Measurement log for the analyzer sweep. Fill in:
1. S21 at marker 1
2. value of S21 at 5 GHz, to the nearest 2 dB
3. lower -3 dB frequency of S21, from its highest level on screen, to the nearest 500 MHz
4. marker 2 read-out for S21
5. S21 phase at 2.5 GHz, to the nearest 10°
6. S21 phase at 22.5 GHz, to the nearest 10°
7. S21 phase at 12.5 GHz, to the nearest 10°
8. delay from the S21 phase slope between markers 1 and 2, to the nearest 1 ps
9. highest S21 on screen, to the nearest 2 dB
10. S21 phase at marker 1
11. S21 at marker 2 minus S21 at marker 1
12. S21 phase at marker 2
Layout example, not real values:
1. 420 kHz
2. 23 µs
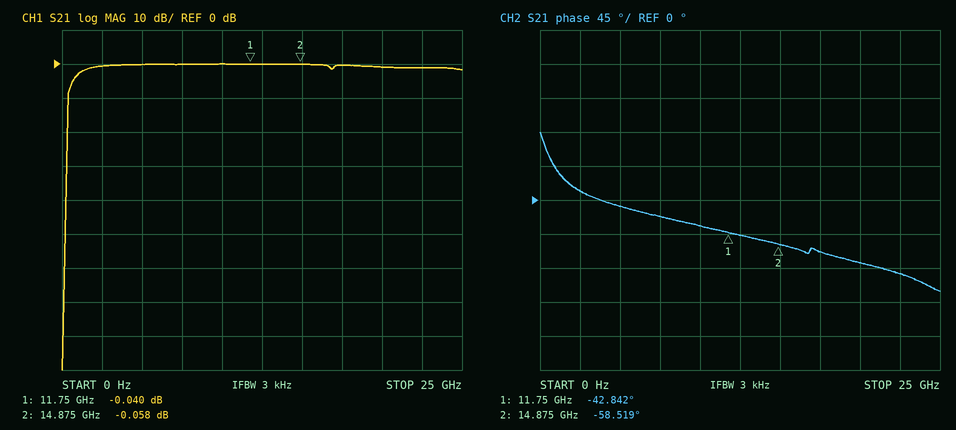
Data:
1. -0.040 dB
2. 0 dB
3. 1.0 GHz
4. -0.058 dB
5. 10°
6. -100°
7. -50°
8. 14 ps
9. 0 dB
10. -42.842°
11. -0.018 dB
12. -58.519°
